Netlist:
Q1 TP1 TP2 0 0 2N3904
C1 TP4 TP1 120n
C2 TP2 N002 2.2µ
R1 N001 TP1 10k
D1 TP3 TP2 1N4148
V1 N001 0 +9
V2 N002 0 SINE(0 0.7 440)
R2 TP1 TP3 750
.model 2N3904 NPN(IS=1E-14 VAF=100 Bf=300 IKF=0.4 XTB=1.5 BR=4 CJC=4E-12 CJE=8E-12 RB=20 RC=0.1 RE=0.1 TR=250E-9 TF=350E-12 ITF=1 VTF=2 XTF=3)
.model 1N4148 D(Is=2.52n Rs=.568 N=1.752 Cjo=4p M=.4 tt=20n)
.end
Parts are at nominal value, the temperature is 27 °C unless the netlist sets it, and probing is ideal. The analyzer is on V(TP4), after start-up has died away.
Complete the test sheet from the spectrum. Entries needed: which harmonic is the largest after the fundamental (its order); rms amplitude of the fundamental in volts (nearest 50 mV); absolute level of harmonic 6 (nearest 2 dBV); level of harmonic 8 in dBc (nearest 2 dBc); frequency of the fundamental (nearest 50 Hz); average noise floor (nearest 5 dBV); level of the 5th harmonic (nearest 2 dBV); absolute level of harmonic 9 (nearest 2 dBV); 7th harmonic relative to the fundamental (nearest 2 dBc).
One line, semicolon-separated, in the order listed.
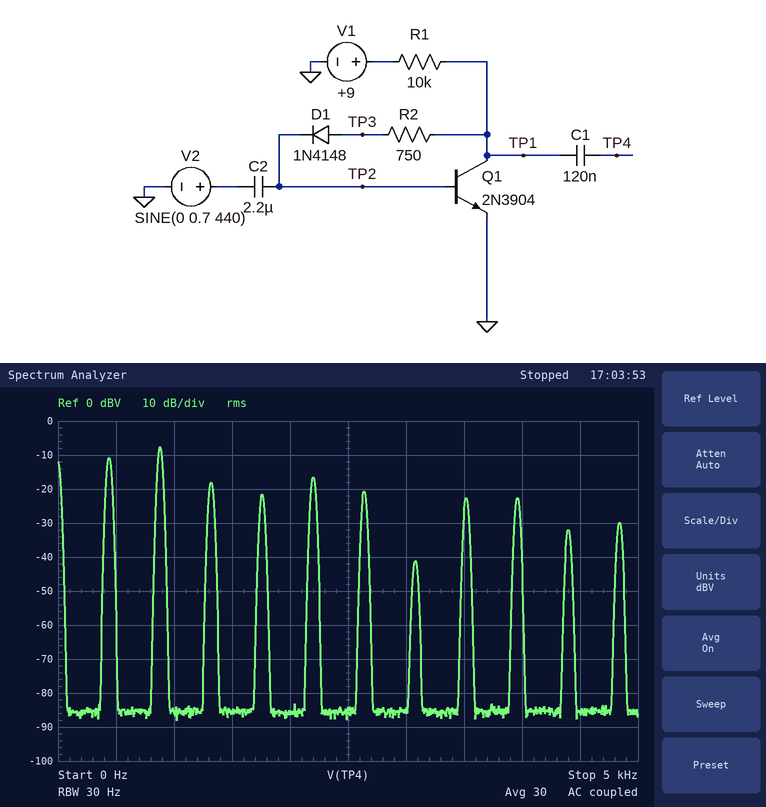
2; 300 mV; -20 dBV; -12 dBc; 450 Hz; -85 dBV; -16 dBV; -22 dBV; -30 dBc
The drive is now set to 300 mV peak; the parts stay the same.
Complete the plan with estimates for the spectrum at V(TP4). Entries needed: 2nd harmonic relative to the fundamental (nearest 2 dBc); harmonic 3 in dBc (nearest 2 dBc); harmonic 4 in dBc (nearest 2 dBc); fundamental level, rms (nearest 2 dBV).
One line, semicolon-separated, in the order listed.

-10 dBc; -12 dBc; -12 dBc; -4 dBV
